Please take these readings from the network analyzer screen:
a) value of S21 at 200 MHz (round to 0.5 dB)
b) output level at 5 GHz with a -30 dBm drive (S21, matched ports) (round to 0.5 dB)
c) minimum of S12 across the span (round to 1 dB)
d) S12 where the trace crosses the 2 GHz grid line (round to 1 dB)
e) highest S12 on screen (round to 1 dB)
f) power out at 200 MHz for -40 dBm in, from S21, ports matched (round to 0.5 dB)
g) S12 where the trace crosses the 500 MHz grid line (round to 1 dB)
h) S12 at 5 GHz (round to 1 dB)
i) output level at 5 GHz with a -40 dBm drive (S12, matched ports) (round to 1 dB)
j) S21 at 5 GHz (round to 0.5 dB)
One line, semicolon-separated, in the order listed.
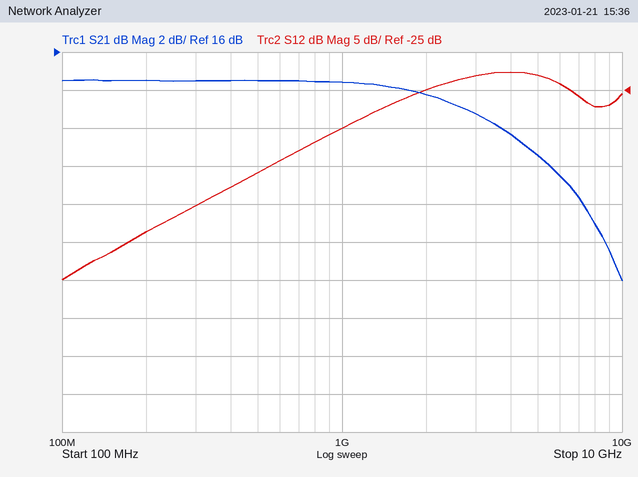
14.5 dB; -19.5 dBm; -50 dB; -25 dB; -23 dB; -25.5 dBm; -36 dB; -23 dB; -63 dBm; 10.5 dB
